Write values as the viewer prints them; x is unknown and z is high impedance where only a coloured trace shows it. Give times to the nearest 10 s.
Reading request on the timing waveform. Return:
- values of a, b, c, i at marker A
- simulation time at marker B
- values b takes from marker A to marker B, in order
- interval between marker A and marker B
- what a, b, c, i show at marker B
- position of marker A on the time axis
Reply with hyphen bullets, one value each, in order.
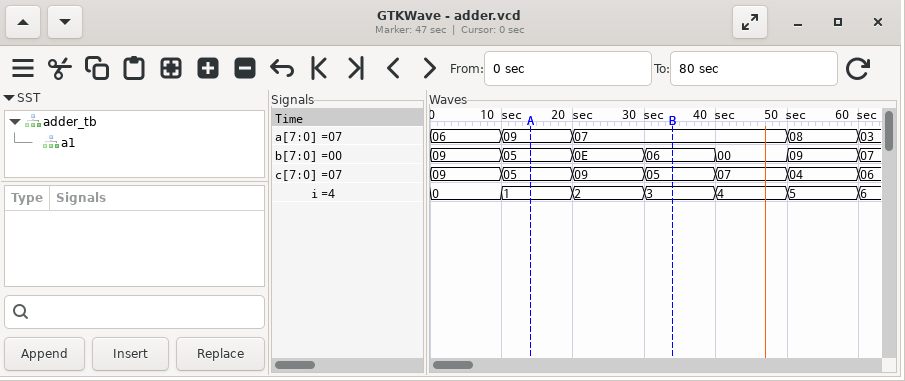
- a=09, b=05, c=05, i=1
- 30 s
- 05, 0E, 06
- 20 s
- a=07, b=06, c=05, i=3
- 10 s
